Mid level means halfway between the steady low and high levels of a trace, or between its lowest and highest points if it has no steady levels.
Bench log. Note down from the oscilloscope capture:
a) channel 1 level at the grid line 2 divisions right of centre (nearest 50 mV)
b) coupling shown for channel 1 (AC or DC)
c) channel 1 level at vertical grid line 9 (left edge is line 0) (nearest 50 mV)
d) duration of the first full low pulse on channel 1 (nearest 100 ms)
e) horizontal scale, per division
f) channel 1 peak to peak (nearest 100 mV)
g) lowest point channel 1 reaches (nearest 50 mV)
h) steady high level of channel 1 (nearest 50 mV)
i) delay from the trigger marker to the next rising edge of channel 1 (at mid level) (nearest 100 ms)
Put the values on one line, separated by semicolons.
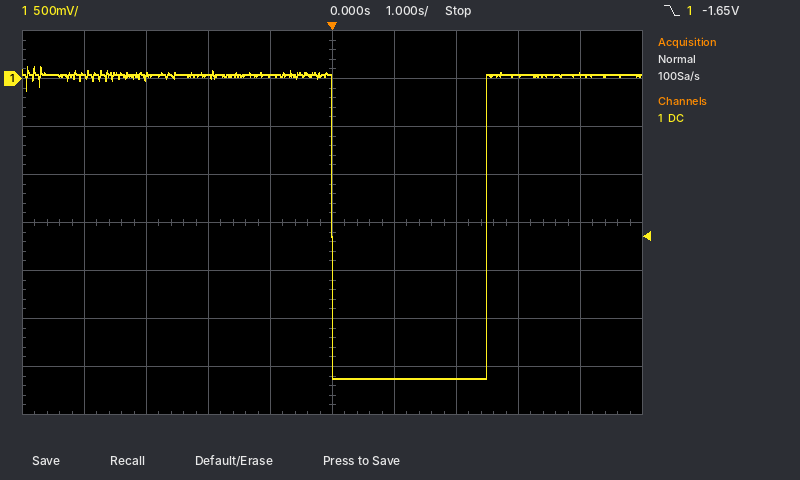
-3.10 V; DC; 50 mV; 2.5 s; 1 s; 3.20 V; -3.10 V; 50 mV; 2.5 s
